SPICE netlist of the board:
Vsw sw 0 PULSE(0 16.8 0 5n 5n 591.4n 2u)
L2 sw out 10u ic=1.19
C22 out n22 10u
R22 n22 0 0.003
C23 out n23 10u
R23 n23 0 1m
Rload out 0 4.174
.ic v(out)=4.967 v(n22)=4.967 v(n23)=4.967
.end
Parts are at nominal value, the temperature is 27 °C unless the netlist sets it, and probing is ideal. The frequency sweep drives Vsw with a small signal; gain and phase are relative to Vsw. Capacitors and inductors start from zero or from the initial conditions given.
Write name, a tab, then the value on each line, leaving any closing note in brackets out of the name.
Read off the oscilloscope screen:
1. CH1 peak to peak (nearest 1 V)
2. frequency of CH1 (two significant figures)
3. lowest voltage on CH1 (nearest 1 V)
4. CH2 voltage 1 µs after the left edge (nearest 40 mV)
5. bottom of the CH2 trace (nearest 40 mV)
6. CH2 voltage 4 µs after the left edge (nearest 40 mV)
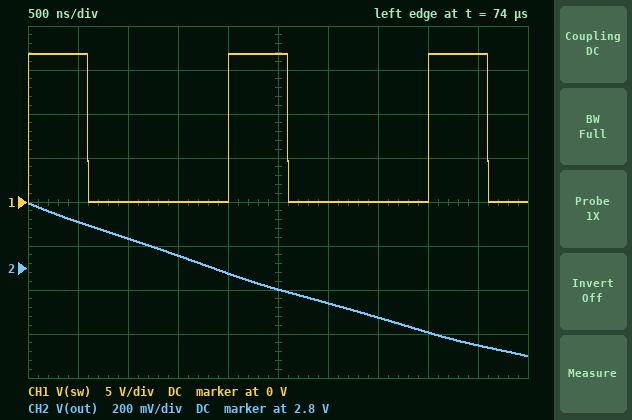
CH1 peak to peak	17 V
frequency of CH1	500 kHz
lowest voltage on CH1	0 V
CH2 voltage 1 µs after the left edge	2.92 V
bottom of the CH2 trace	2.40 V
CH2 voltage 4 µs after the left edge	2.52 V
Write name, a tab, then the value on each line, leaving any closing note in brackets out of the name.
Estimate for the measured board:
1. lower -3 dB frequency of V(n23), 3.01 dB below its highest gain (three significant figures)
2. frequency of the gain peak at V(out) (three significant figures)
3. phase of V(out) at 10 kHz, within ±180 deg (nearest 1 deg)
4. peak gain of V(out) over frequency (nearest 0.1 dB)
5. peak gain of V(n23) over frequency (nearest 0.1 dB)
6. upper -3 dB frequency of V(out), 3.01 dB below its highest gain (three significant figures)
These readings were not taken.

lower -3 dB frequency of V(n23), 3.01 dB below its highest gain	10.3 kHz
frequency of the gain peak at V(out)	11.2 kHz
phase of V(out) at 10 kHz, within ±180 deg	-36 deg
peak gain of V(out) over frequency	15.4 dB
peak gain of V(n23) over frequency	-47.7 dB
upper -3 dB frequency of V(out), 3.01 dB below its highest gain	12.1 kHz
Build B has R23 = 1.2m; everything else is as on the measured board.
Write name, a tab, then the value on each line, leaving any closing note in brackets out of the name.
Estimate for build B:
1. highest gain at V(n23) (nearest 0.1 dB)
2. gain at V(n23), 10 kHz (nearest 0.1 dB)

highest gain at V(n23)	-46.1 dB
gain at V(n23), 10 kHz	-50.7 dB
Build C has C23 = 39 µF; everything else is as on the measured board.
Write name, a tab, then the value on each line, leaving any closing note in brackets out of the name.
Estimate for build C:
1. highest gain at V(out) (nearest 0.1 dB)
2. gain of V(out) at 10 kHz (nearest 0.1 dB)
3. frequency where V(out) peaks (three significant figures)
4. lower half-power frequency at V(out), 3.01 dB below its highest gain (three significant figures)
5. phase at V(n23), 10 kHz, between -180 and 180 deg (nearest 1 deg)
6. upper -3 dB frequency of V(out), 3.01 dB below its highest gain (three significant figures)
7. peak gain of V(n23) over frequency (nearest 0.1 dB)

highest gain at V(out)	19.2 dB
gain of V(out) at 10 kHz	0.5 dB
frequency where V(out) peaks	7.17 kHz
lower half-power frequency at V(out), 3.01 dB below its highest gain	6.76 kHz
phase at V(n23), 10 kHz, between -180 and 180 deg	-81 deg
upper -3 dB frequency of V(out), 3.01 dB below its highest gain	7.55 kHz
peak gain of V(n23) over frequency	-35.9 dB
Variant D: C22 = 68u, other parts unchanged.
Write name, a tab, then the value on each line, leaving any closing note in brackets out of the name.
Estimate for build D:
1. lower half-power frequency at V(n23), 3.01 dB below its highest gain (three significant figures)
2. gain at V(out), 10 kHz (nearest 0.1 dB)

lower half-power frequency at V(n23), 3.01 dB below its highest gain	5.44 kHz
gain at V(out), 10 kHz	-6.4 dB
